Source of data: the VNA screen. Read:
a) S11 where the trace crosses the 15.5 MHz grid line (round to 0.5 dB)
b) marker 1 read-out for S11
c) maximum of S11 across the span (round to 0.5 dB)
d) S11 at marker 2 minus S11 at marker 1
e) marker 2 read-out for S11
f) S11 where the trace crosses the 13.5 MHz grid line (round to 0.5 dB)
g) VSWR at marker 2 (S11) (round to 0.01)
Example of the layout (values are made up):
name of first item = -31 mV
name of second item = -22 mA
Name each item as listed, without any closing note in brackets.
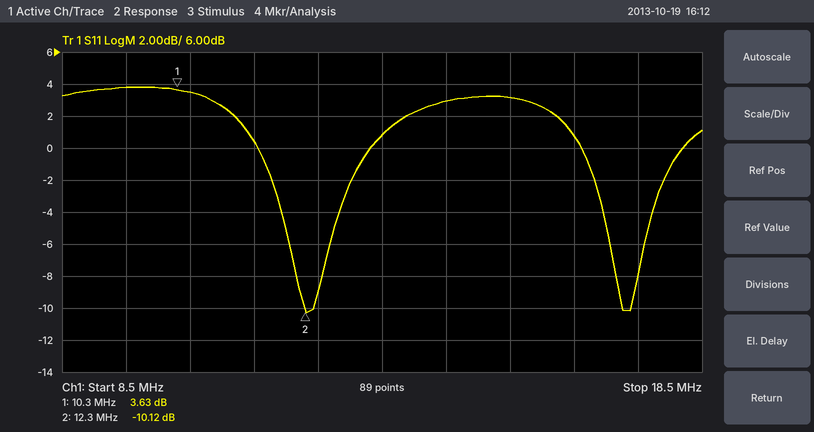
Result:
S11 where the trace crosses the 15.5 MHz grid line = 3.0 dB
marker 1 read-out for S11 = 3.63 dB
maximum of S11 across the span = 4.0 dB
S11 at marker 2 minus S11 at marker 1 = -13.75 dB
marker 2 read-out for S11 = -10.12 dB
S11 where the trace crosses the 13.5 MHz grid line = 1.0 dB
VSWR at marker 2 (S11) = 1.91
